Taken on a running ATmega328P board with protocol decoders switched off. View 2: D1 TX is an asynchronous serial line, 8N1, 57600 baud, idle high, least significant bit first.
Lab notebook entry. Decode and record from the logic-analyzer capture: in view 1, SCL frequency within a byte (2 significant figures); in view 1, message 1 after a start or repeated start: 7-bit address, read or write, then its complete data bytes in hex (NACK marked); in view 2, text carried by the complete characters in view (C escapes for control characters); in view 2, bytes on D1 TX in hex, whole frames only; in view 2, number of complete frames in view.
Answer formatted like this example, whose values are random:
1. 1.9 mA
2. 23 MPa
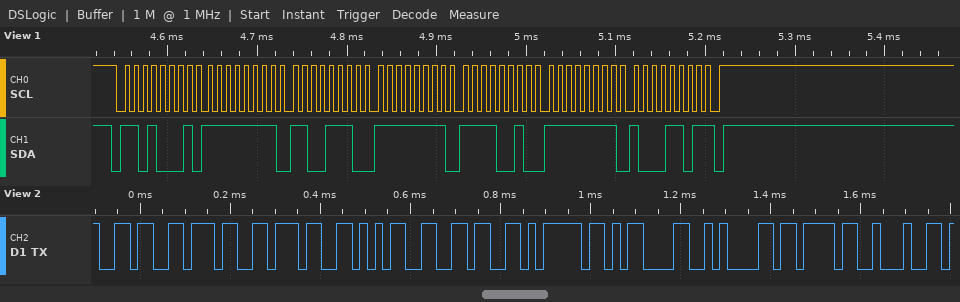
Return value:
1. 100 kHz
2. 0x68 read: FF CE FF F2 FF 8D NACK
3. "67756}\r\n{\""
4. 36 37 37 35 36 7D 0D 0A 7B 22
5. 10
